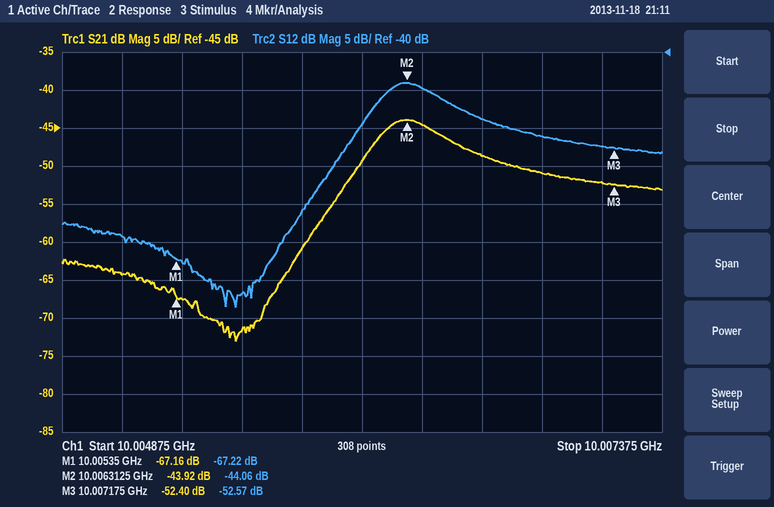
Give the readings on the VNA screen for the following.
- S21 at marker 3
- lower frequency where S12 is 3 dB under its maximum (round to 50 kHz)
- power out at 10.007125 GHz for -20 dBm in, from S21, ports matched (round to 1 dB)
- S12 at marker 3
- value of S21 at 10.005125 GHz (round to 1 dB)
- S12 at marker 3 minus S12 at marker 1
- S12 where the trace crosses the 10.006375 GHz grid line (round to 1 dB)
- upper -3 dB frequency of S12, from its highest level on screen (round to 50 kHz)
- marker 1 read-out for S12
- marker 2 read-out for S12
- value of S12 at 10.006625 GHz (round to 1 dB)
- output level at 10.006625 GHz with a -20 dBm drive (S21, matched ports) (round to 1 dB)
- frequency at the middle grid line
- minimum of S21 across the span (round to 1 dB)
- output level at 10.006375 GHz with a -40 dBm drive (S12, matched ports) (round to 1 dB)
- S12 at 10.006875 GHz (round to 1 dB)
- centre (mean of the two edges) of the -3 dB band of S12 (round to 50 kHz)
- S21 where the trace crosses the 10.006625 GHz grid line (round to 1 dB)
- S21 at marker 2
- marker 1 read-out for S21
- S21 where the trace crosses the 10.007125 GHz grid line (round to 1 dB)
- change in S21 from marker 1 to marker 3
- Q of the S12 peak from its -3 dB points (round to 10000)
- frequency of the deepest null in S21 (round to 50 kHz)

-52.40 dB
10.00620 GHz
-72 dBm
-52.57 dB
-64 dB
14.65 dB
-45 dB
10.00650 GHz
-67.22 dB
-44.06 dB
-49 dB
-69 dBm
10.006125 GHz
-73 dB
-85 dBm
-51 dB
10.00635 GHz
-49 dB
-43.92 dB
-67.16 dB
-52 dB
14.76 dB
30000
10.00560 GHz
